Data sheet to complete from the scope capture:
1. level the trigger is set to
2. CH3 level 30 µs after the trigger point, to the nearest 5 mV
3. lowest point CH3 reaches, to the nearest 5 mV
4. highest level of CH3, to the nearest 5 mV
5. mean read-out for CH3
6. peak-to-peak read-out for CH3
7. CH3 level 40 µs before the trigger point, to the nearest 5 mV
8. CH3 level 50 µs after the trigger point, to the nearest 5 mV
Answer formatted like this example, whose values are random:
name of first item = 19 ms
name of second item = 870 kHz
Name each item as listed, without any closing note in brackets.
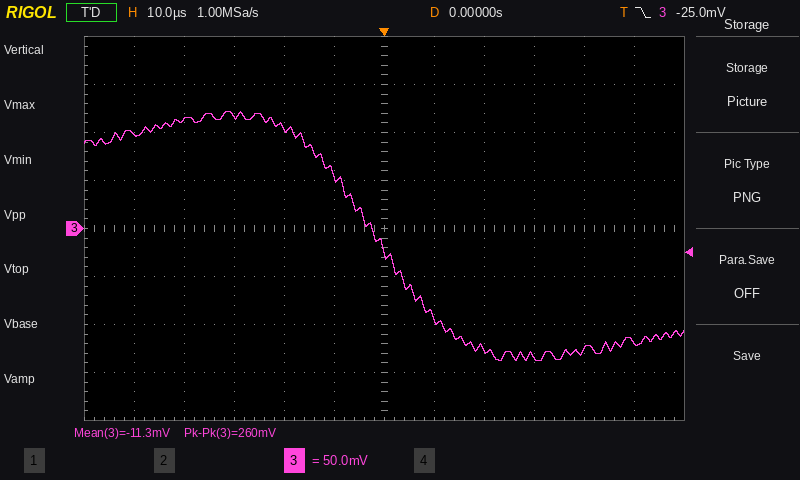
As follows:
level the trigger is set to = -25.0 mV
CH3 level 30 µs after the trigger point, to the nearest 5 mV = -135 mV
lowest point CH3 reaches, to the nearest 5 mV = -140 mV
highest level of CH3, to the nearest 5 mV = 120 mV
mean read-out for CH3 = -11.3 mV
peak-to-peak read-out for CH3 = 260 mV
CH3 level 40 µs before the trigger point, to the nearest 5 mV = 115 mV
CH3 level 50 µs after the trigger point, to the nearest 5 mV = -120 mV
